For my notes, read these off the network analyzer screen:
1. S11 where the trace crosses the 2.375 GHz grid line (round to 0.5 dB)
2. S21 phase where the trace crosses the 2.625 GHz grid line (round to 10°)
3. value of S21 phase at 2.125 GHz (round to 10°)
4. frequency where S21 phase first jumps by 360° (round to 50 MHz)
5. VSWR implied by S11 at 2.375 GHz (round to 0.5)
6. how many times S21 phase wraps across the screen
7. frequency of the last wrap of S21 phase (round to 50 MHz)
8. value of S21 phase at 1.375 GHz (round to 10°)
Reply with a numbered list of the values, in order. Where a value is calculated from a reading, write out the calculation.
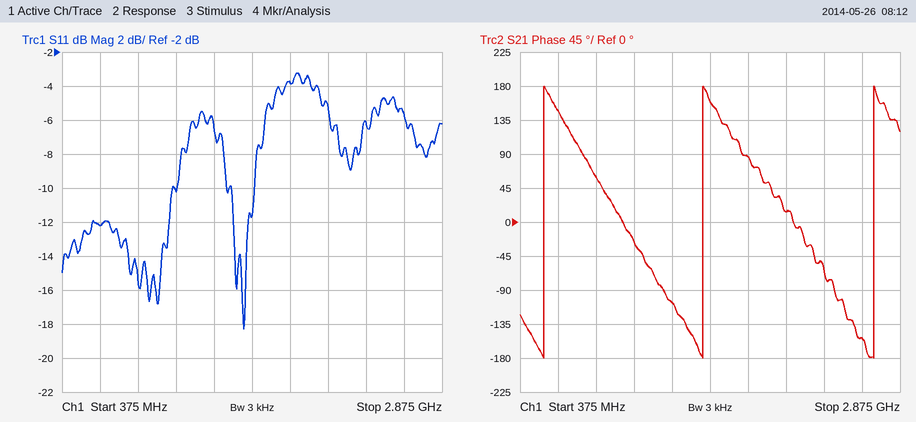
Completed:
1. -6.0 dB
2. -150°
3. 10°
4. 550 MHz
5. |Γ| = 10^(-6/20) = 0.5012; VSWR = (1 + 0.5012)/(1 − 0.5012) ≈ 3.0
6. 3
7. 2.70 GHz
8. -110°
